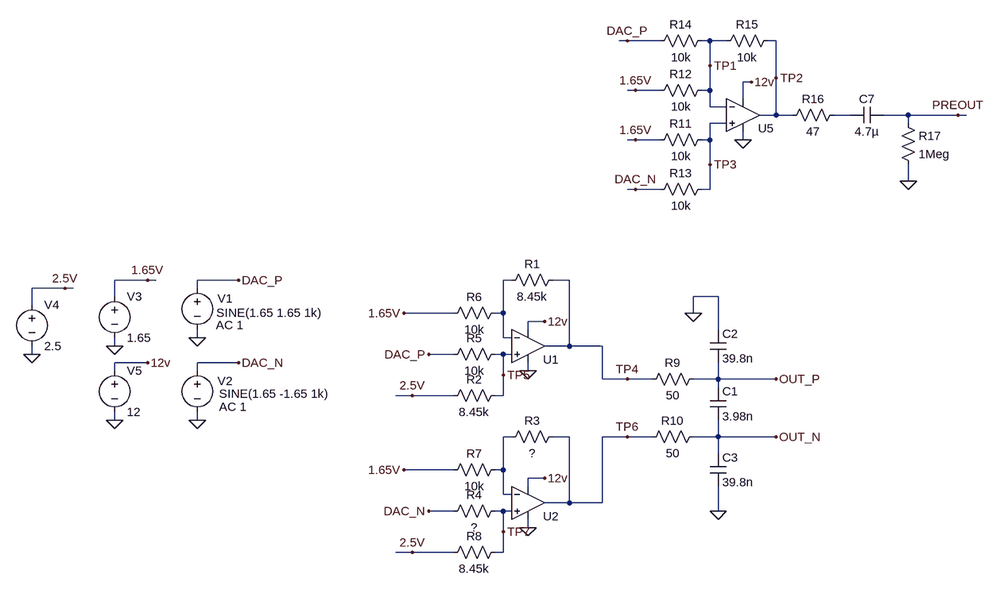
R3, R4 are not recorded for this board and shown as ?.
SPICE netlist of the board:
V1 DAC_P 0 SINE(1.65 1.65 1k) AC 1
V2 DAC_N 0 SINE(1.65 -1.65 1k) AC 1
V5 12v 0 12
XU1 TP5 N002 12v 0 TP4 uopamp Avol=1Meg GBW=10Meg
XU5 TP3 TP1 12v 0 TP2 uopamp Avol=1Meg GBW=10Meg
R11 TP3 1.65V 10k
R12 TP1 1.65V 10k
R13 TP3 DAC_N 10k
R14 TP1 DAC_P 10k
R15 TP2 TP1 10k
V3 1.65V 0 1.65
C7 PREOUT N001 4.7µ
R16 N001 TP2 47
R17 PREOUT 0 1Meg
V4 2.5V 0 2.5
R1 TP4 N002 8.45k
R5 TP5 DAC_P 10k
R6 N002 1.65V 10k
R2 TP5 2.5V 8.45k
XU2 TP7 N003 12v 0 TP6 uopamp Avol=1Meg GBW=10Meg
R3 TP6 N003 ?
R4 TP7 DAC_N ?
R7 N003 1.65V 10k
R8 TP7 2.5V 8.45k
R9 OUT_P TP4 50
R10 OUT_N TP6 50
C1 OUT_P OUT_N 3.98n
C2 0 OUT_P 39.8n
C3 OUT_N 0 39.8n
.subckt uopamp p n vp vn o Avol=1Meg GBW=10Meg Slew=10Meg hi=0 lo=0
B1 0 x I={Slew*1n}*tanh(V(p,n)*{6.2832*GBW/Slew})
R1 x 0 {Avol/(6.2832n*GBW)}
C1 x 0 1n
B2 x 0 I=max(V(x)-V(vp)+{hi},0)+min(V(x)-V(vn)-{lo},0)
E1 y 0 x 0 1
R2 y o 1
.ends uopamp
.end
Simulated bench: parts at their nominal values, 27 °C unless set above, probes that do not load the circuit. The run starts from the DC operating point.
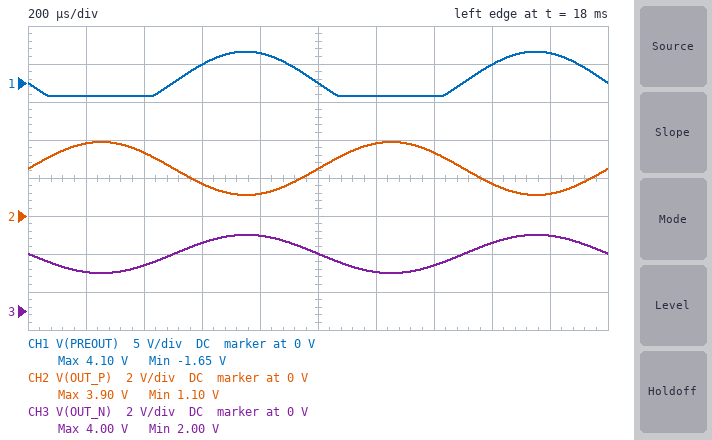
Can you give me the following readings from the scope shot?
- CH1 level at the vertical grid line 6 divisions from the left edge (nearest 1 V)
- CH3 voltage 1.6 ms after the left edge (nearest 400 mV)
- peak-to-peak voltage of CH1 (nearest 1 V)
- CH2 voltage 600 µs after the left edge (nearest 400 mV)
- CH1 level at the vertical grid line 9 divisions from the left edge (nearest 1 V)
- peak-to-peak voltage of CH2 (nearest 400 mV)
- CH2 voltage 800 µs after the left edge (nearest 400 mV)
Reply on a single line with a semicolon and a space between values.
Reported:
-2 V; 3.6 V; 6 V; 1.6 V; 4 V; 2.8 V; 1.2 V
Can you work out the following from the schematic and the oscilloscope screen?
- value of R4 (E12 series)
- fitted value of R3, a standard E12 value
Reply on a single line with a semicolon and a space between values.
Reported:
22 kΩ; 12 kΩ
